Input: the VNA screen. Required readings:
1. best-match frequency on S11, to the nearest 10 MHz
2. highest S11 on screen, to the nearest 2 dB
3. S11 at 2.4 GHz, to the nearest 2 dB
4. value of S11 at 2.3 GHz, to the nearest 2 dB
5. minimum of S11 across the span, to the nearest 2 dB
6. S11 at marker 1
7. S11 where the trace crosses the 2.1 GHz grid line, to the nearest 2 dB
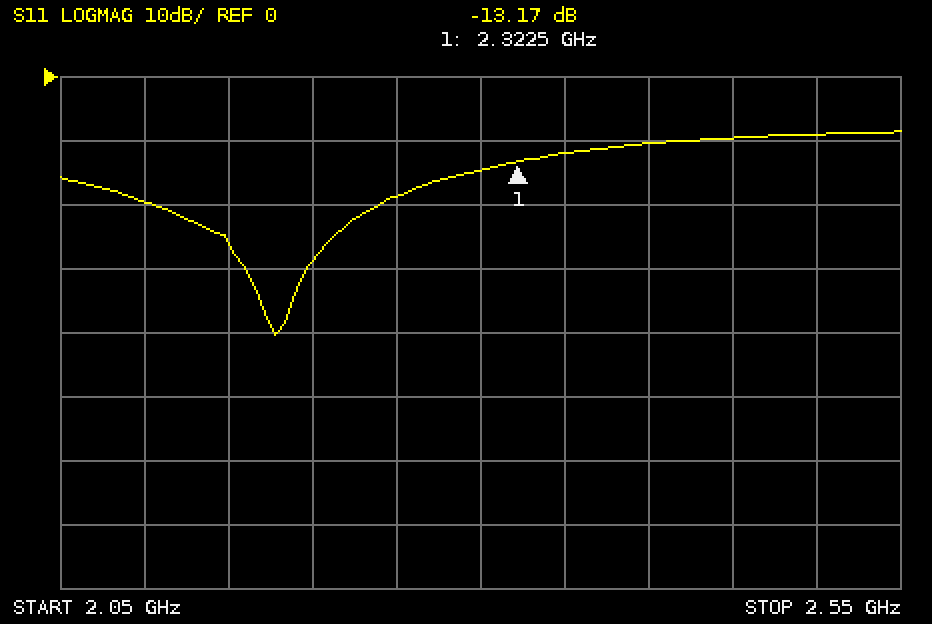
2.18 GHz
-8 dB
-10 dB
-14 dB
-40 dB
-13.17 dB
-20 dB
